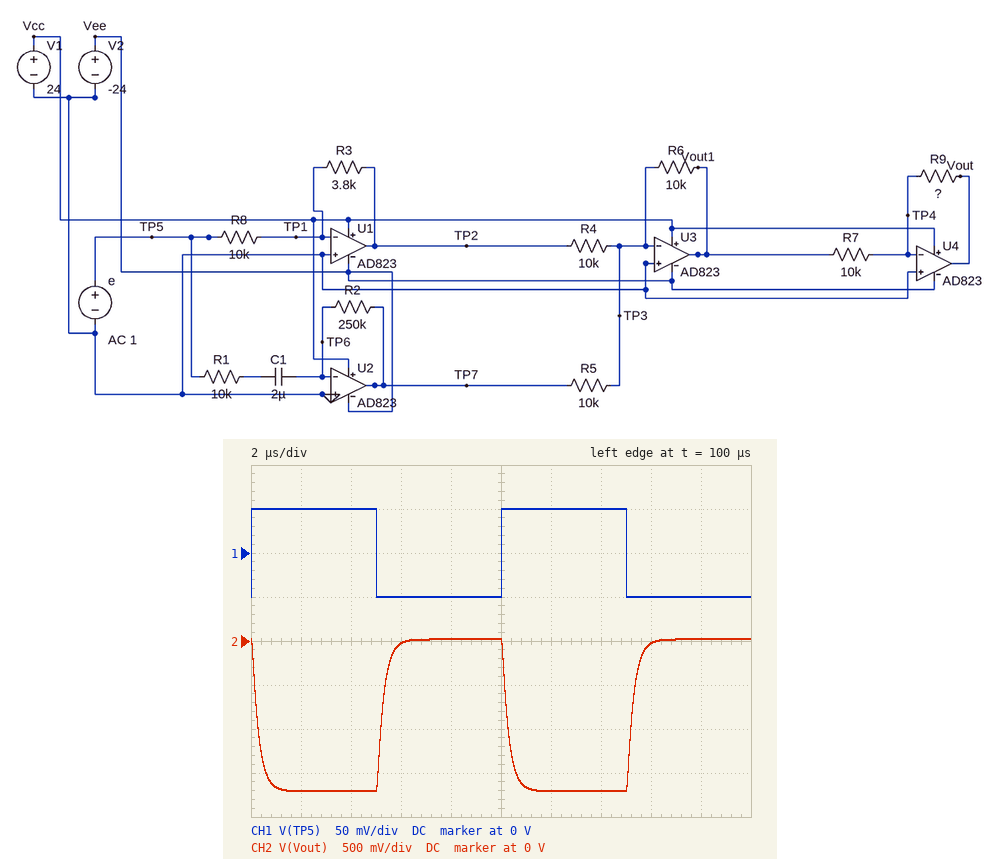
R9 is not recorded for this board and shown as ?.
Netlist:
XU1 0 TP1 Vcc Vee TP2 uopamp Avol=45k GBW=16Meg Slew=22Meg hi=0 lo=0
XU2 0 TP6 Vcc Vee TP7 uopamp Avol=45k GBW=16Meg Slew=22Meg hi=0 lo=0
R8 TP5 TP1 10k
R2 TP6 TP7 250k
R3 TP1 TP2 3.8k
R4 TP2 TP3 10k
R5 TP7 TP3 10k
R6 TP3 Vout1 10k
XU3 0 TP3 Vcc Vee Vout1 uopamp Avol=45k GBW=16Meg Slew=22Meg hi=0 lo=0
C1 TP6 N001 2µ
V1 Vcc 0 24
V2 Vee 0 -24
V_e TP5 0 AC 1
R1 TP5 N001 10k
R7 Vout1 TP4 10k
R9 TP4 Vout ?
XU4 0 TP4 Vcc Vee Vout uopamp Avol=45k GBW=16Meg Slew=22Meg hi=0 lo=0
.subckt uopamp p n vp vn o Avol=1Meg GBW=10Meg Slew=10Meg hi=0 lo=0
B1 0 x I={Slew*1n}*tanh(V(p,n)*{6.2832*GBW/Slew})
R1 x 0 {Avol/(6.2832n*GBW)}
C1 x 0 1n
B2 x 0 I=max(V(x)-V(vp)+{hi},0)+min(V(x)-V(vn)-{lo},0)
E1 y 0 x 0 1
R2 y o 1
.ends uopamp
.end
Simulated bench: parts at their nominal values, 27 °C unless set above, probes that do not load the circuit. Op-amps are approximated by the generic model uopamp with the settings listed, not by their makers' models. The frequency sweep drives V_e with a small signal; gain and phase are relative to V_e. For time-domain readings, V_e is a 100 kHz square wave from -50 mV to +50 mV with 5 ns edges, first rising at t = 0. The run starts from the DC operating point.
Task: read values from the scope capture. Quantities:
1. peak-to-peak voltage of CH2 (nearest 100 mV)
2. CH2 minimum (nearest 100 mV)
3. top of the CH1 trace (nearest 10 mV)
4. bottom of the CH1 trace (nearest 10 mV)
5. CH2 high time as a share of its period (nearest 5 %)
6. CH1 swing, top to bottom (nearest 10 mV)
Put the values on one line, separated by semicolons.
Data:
1.7 V; -1.7 V; 50 mV; -50 mV; 50 %; 100 mV
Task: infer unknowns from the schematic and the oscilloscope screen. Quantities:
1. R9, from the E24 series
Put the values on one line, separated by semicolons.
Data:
6.8 kΩ
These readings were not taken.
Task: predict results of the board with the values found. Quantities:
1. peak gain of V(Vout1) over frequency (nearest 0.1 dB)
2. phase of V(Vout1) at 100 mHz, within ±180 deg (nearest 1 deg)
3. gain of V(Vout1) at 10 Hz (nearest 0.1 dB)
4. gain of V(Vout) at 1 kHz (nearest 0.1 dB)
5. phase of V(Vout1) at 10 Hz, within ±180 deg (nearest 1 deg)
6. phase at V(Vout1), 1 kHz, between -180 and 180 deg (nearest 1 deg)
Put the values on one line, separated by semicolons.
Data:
28.1 dB; 39 deg; 26.0 dB; 24.7 dB; 38 deg; 0 deg
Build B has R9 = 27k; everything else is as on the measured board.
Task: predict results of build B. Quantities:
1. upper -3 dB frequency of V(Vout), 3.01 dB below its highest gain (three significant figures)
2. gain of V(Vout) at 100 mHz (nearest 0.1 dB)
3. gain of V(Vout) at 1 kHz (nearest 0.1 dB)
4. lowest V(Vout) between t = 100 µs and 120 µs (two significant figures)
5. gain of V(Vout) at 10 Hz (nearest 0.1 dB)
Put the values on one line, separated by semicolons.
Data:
597 kHz; 2.5 dB; 36.7 dB; -6.8 V; 34.6 dB
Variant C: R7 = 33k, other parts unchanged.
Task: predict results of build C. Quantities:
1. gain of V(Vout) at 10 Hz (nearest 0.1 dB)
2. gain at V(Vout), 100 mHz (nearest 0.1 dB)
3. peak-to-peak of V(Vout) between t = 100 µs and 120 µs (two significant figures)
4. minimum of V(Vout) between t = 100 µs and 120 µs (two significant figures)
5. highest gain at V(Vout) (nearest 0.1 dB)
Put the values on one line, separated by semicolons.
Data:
12.2 dB; -19.8 dB; 520 mV; -520 mV; 14.4 dB
